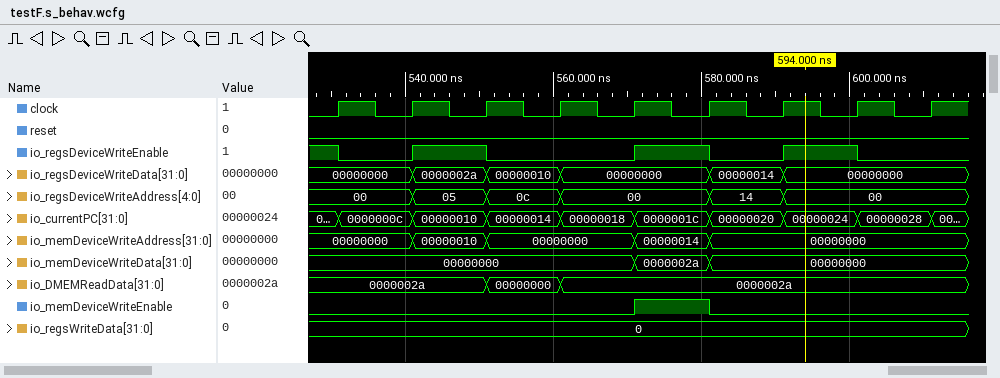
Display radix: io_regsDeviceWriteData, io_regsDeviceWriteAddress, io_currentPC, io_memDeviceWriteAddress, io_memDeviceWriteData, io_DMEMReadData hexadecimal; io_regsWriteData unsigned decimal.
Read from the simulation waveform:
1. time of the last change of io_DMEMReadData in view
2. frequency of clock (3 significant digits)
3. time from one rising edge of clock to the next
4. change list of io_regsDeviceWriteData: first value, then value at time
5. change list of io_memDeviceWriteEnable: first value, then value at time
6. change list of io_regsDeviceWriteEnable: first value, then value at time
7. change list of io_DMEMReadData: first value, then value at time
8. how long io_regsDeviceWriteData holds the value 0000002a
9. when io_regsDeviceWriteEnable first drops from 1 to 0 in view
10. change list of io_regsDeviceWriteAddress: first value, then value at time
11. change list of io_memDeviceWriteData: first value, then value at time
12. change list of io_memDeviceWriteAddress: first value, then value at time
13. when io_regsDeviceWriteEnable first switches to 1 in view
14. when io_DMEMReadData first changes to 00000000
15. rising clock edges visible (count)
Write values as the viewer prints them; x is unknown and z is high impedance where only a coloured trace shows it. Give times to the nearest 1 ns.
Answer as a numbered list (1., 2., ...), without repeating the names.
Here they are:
1. 561 ns
2. 100 MHz
3. 10 ns
4. 00000000, 0000002a at 541 ns, 00000010 at 551 ns, 00000000 at 561 ns, 00000014 at 581 ns, 00000000 at 591 ns
5. 0, 1 at 571 ns, 0 at 581 ns
6. 1, 0 at 531 ns, 1 at 541 ns, 0 at 551 ns, 1 at 571 ns, 0 at 581 ns, 1 at 591 ns, 0 at 601 ns
7. 0000002a, 00000000 at 551 ns, 0000002a at 561 ns
8. 10 ns
9. 531 ns
10. 00, 05 at 541 ns, 0c at 551 ns, 00 at 561 ns, 14 at 581 ns, 00 at 591 ns
11. 00000000, 0000002a at 571 ns, 00000000 at 581 ns
12. 00000000, 00000010 at 541 ns, 00000000 at 551 ns, 00000014 at 571 ns, 00000000 at 581 ns
13. 541 ns
14. 551 ns
15. 9
